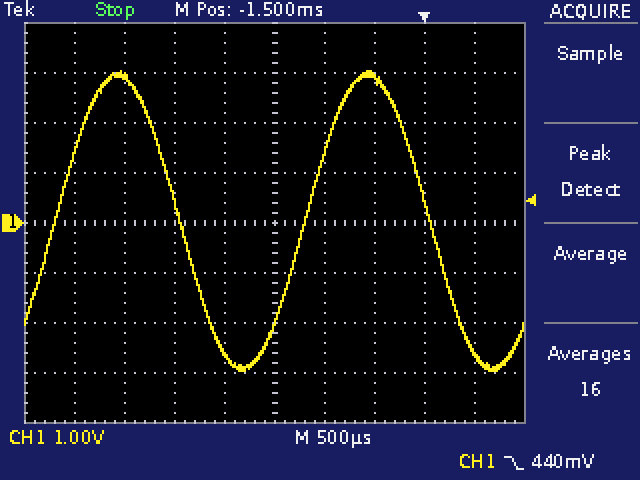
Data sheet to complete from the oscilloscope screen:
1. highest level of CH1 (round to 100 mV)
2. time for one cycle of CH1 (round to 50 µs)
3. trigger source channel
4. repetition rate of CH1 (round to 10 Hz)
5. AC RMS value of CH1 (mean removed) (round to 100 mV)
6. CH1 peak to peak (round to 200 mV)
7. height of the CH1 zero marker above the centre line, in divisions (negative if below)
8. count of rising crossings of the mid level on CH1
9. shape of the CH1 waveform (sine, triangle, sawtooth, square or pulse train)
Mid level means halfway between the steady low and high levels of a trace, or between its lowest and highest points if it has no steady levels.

3.0 V
2.50 ms
CH1
400 Hz
2.1 V
6.0 V
0.0 div
2
sine
